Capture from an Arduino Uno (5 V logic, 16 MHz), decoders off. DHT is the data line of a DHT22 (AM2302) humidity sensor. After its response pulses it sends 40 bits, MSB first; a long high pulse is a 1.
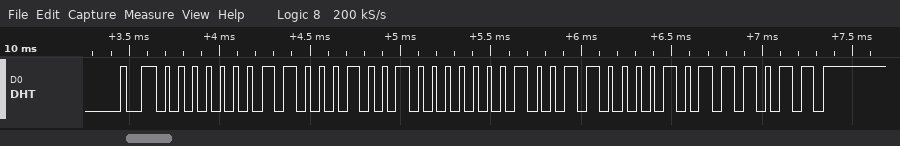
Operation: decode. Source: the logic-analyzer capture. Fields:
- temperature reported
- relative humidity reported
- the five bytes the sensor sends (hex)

30.4 °C
39.3 %
01 89 01 30 BB
